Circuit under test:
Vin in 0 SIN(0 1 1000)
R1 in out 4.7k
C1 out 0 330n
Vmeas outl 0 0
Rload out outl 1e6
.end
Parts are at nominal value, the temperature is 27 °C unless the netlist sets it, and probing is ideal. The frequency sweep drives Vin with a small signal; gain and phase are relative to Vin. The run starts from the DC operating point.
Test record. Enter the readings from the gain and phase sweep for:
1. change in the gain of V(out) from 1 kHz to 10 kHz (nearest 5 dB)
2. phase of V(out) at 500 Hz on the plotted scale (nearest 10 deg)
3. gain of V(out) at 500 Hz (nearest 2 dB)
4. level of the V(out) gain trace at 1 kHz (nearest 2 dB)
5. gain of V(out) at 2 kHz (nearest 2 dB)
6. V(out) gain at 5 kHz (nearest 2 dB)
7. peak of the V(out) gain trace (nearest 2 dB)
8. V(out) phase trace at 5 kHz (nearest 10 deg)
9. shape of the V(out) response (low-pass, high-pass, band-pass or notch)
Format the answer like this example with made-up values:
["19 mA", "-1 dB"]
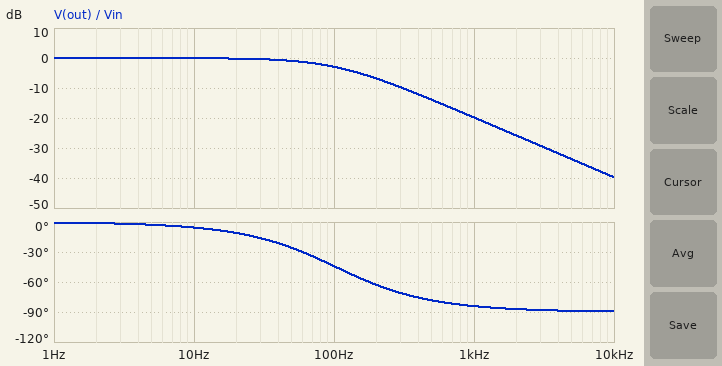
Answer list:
["-20 dB", "-80 deg", "-14 dB", "-20 dB", "-26 dB", "-34 dB", "0 dB", "-90 deg", "low-pass"]
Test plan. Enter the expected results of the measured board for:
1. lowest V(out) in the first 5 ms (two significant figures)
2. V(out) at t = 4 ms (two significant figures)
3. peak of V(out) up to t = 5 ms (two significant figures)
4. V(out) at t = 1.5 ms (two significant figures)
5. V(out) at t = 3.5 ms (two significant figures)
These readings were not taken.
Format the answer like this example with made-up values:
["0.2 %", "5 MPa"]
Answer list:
["-98 mV", "-94 mV", "180 mV", "140 mV", "110 mV"]
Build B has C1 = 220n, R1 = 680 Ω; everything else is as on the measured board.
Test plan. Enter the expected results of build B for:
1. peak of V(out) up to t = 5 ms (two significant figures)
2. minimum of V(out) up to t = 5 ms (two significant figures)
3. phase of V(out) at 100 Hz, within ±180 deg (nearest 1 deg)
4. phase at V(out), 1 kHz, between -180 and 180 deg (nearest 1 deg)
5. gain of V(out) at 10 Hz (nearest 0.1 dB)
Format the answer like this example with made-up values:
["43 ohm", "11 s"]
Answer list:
["770 mV", "-730 mV", "-5 deg", "-43 deg", "0 dB"]
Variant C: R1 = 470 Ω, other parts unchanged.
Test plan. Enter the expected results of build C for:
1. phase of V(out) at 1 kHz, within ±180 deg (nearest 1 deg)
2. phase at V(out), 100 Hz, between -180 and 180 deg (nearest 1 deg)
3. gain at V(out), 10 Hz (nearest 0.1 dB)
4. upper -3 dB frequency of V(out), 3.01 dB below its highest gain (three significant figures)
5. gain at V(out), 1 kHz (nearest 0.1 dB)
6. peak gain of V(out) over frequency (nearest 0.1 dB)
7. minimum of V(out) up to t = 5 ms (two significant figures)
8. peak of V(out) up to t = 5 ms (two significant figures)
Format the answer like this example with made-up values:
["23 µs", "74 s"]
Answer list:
["-44 deg", "-6 deg", "0 dB", "1.03 kHz", "-2.9 dB", "0 dB", "-720 mV", "760 mV"]
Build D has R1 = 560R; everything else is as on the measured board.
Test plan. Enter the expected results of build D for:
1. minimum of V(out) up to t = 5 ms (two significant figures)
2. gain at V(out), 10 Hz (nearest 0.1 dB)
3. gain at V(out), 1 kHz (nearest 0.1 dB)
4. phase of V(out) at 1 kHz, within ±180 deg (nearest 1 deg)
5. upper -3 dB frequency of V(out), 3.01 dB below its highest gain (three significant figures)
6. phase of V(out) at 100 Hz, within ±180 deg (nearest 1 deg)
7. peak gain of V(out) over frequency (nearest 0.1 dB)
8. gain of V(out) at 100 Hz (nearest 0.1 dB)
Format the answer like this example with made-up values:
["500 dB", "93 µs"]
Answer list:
["-650 mV", "0 dB", "-3.7 dB", "-49 deg", "862 Hz", "-7 deg", "0 dB", "-0.1 dB"]
